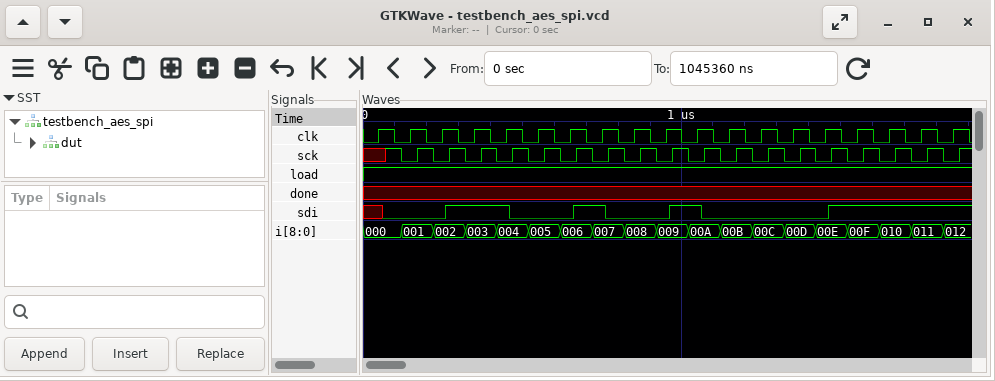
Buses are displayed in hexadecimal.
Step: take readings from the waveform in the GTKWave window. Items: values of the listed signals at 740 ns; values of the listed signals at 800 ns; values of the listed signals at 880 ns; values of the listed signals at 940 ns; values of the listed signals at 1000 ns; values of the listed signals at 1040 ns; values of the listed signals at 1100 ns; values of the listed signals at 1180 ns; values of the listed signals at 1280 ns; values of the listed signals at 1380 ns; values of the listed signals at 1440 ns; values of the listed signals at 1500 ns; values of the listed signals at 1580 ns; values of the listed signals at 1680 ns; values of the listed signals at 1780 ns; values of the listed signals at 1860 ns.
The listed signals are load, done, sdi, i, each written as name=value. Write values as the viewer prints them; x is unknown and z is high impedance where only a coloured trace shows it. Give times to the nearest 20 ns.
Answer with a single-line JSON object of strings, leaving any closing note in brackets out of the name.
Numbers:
{"values of the listed signals at 740 ns": "load=1, done=x, sdi=1, i=007", "values of the listed signals at 800 ns": "load=1, done=x, sdi=0, i=007", "values of the listed signals at 880 ns": "load=1, done=x, sdi=0, i=008", "values of the listed signals at 940 ns": "load=1, done=x, sdi=0, i=009", "values of the listed signals at 1000 ns": "load=1, done=x, sdi=1, i=009", "values of the listed signals at 1040 ns": "load=1, done=x, sdi=1, i=00A", "values of the listed signals at 1100 ns": "load=1, done=x, sdi=0, i=00A", "values of the listed signals at 1180 ns": "load=1, done=x, sdi=0, i=00B", "values of the listed signals at 1280 ns": "load=1, done=x, sdi=0, i=00C", "values of the listed signals at 1380 ns": "load=1, done=x, sdi=0, i=00D", "values of the listed signals at 1440 ns": "load=1, done=x, sdi=0, i=00E", "values of the listed signals at 1500 ns": "load=1, done=x, sdi=1, i=00E", "values of the listed signals at 1580 ns": "load=1, done=x, sdi=1, i=00F", "values of the listed signals at 1680 ns": "load=1, done=x, sdi=1, i=010", "values of the listed signals at 1780 ns": "load=1, done=x, sdi=1, i=011", "values of the listed signals at 1860 ns": "load=1, done=x, sdi=1, i=012"}
